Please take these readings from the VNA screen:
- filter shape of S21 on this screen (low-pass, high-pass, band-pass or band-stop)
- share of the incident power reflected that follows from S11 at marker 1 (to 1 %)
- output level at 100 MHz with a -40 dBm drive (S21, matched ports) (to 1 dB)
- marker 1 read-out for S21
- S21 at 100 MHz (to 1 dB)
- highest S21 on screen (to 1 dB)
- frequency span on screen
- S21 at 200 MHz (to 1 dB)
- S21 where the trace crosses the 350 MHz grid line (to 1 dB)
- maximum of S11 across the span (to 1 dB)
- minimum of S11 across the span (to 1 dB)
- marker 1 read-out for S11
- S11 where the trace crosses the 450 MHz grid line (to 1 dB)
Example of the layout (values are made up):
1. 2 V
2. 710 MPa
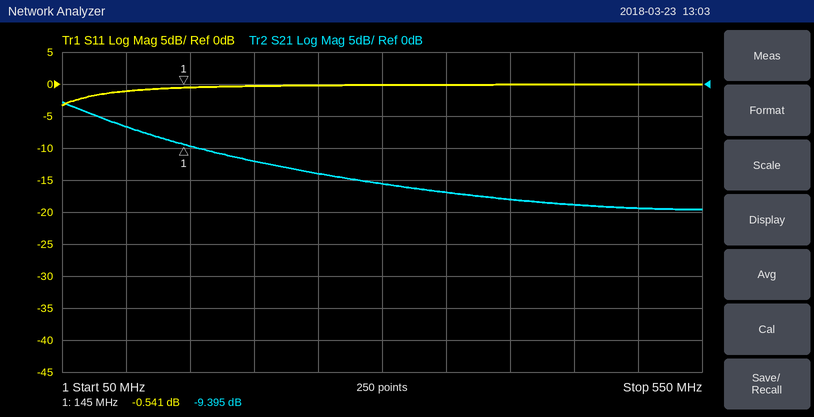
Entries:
1. low-pass
2. 88 %
3. -47 dBm
4. -9.395 dB
5. -7 dB
6. -3 dB
7. 500 MHz
8. -12 dB
9. -17 dB
10. 0 dB
11. -3 dB
12. -0.541 dB
13. 0 dB
